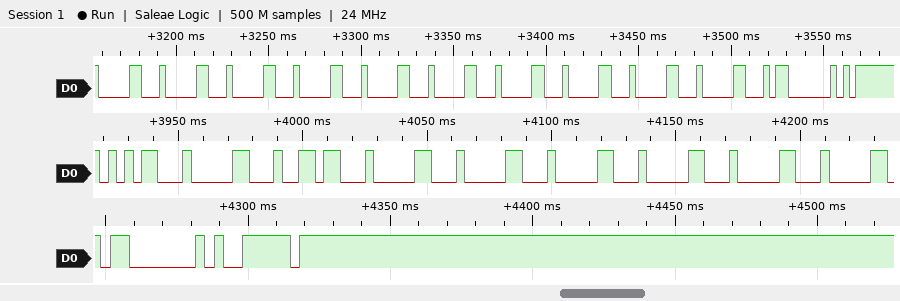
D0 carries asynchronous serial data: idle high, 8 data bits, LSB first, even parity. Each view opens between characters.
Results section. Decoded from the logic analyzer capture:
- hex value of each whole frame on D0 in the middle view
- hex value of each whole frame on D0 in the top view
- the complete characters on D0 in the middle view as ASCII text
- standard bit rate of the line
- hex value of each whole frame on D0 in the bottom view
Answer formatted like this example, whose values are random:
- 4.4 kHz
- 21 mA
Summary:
- 35, 30, 36, 30, 30, 30, 30, 30
- 30, 30, 30, 30, 30, 30, 30, 30, 30, 30, 03
- "50600000"
- 300 baud
- 03, F9
